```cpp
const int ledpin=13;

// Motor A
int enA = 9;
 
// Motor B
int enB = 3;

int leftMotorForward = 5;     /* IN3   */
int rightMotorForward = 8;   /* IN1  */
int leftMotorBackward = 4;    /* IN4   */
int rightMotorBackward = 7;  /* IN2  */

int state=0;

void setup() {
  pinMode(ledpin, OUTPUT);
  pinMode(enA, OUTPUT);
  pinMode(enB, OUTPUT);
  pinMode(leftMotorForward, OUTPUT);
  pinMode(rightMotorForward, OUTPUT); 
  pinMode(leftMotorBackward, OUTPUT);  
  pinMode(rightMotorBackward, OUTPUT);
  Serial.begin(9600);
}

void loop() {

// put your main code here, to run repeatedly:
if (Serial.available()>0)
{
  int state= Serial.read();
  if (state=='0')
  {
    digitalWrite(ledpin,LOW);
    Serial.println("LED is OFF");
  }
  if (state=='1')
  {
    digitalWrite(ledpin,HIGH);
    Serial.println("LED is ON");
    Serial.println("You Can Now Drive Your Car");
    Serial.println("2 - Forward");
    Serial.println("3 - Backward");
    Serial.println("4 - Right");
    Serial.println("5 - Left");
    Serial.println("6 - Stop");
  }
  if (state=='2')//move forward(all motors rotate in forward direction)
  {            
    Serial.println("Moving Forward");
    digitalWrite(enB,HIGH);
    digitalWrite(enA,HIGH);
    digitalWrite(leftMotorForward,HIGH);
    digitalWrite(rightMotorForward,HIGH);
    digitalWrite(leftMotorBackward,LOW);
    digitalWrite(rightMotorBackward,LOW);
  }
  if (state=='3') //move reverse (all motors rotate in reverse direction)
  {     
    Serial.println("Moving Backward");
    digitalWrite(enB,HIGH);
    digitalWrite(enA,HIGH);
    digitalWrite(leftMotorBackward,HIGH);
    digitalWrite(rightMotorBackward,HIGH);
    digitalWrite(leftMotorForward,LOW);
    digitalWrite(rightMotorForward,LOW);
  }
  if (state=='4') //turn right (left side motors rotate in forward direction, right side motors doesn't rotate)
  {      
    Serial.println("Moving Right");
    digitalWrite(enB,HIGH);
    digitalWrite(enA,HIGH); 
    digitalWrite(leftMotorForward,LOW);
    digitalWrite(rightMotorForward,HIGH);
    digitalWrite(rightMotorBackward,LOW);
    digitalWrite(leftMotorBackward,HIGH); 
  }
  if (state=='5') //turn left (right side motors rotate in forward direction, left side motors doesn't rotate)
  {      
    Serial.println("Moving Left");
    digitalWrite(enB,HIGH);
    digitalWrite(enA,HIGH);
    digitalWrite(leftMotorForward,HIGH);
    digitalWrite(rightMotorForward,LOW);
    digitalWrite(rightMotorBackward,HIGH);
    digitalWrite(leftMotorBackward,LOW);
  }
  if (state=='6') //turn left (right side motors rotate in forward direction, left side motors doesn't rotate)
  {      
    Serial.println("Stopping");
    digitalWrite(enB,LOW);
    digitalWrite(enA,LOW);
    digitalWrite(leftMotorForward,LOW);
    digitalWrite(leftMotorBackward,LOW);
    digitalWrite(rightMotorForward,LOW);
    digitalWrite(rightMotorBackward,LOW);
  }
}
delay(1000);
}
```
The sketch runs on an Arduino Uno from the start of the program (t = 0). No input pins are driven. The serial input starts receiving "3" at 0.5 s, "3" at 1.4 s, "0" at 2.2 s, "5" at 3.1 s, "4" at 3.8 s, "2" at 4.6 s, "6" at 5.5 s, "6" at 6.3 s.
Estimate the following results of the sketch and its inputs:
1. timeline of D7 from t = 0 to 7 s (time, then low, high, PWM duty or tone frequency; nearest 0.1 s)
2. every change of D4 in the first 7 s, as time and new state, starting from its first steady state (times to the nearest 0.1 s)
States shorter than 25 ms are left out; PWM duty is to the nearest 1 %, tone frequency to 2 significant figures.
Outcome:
0 s low; 1 s high; 5 s low
0 s low; 1 s high; 4 s low; 5 s high; 6 s low
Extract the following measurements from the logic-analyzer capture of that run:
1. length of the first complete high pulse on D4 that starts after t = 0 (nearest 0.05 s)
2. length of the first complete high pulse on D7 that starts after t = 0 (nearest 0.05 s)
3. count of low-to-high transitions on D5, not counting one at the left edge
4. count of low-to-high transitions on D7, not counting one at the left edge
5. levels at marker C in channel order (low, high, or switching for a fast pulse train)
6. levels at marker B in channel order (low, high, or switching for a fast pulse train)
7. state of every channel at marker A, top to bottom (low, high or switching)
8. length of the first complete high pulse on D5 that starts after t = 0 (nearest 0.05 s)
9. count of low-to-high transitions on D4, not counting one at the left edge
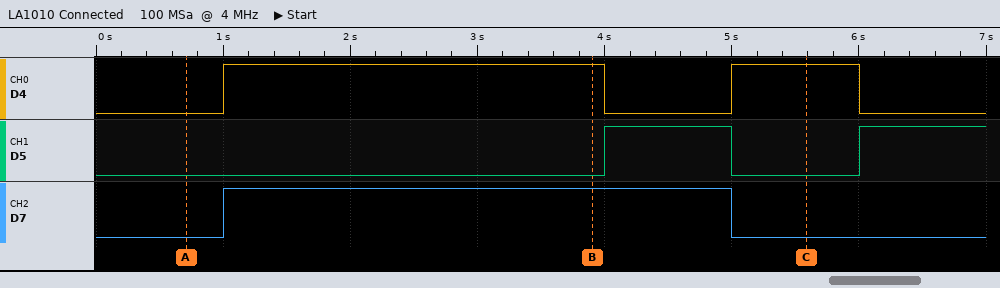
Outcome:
3.00 s
4.00 s
2
1
D4 high, D5 low, D7 low
D4 high, D5 low, D7 high
D4 low, D5 low, D7 low
1.00 s
2
